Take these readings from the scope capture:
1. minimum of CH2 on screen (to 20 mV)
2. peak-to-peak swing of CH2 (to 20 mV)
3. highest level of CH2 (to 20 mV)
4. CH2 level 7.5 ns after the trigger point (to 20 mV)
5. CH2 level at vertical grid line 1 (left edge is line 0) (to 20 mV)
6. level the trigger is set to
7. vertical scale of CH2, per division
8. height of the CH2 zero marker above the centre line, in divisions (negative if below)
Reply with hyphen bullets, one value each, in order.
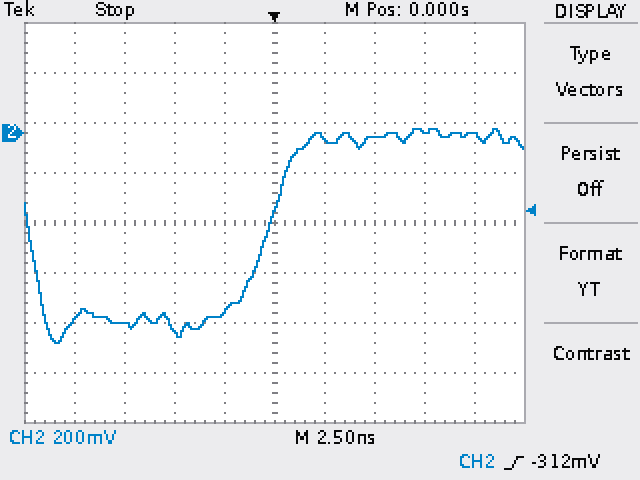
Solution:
- -840 mV
- 860 mV
- 20 mV
- 0 mV
- -740 mV
- -312 mV
- 200 mV
- +1.8 div
